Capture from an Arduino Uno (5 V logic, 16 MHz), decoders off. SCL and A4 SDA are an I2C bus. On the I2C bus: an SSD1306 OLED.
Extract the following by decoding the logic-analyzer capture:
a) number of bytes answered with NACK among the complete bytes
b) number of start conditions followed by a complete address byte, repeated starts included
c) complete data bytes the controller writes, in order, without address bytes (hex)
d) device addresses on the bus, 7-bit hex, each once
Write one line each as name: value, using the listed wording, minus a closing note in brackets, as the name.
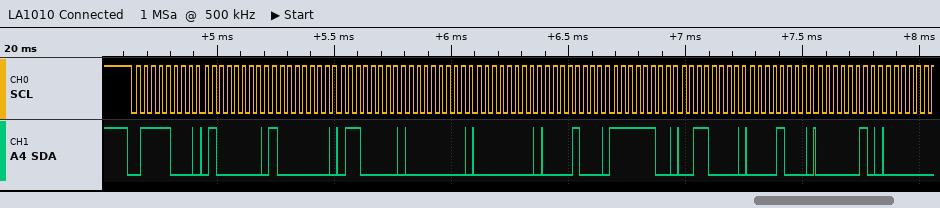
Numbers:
number of bytes answered with NACK among the complete bytes: 0
number of start conditions followed by a complete address byte, repeated starts included: 1
complete data bytes the controller writes, in order, without address bytes: 40 80 60 00 00 08 FC 30 08 02
device addresses on the bus, 7-bit hex, each once: 0x3C
